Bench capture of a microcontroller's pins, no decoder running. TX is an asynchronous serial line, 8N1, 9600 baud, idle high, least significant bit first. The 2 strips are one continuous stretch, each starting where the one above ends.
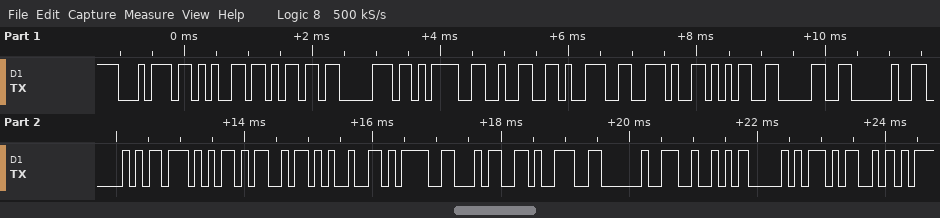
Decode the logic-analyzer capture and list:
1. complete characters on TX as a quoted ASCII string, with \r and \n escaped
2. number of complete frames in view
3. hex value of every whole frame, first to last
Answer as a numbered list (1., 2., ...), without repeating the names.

1. "temp=29.50 PWM%=49 RPM"
2. 22
3. 74 65 6D 70 3D 32 39 2E 35 30 20 50 57 4D 25 3D 34 39 20 52 50 4D
